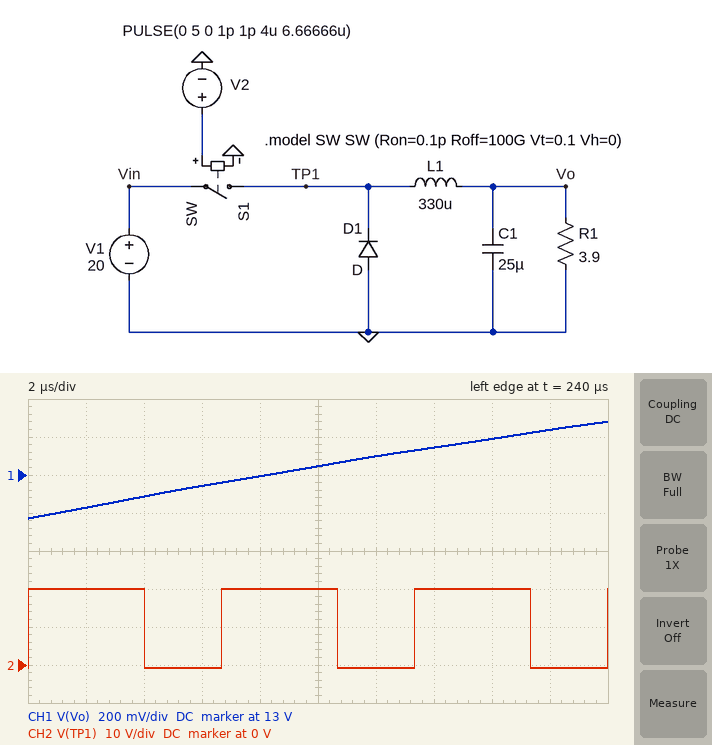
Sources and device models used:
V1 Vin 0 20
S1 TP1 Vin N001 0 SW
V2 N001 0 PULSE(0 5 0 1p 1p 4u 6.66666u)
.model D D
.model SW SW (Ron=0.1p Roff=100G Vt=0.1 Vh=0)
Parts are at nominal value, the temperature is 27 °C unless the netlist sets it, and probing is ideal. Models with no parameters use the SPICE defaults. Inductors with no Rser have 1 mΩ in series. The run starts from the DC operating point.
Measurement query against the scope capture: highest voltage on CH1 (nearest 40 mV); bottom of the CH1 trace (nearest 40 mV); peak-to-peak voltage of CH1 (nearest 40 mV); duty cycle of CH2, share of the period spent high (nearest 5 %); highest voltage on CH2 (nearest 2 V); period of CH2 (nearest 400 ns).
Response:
13.28 V
12.76 V
520 mV
60 %
20 V
6.8 µs
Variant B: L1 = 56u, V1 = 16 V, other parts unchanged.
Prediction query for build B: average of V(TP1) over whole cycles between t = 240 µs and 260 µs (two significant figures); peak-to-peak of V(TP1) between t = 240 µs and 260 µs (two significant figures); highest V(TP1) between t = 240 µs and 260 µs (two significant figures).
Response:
9.3 V
17 V
16 V
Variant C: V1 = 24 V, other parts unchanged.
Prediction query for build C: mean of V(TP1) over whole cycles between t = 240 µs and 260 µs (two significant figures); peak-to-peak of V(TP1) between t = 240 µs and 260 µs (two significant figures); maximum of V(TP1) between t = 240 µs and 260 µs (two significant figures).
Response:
14 V
25 V
24 V
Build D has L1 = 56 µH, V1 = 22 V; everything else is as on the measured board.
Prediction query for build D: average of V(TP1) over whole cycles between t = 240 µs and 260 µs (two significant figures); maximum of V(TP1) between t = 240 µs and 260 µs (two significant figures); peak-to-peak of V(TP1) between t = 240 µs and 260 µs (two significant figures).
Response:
13 V
22 V
23 V
